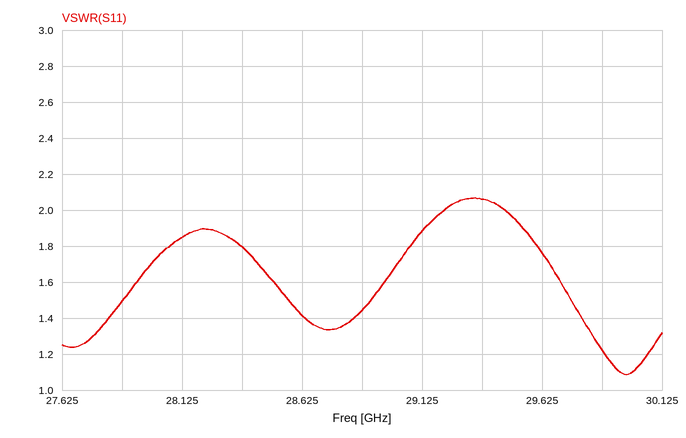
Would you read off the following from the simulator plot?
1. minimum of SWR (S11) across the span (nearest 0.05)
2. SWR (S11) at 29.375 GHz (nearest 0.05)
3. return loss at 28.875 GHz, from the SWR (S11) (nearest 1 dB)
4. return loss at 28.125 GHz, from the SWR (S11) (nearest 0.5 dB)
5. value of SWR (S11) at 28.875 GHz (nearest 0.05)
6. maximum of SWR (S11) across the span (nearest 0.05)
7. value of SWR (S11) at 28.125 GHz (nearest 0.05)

1.10
2.05
15 dB
10.5 dB
1.45
2.05
1.85
